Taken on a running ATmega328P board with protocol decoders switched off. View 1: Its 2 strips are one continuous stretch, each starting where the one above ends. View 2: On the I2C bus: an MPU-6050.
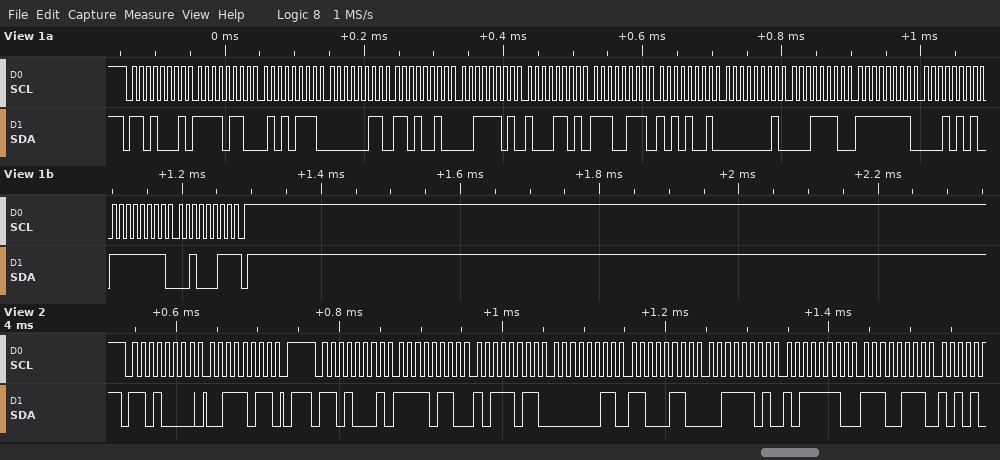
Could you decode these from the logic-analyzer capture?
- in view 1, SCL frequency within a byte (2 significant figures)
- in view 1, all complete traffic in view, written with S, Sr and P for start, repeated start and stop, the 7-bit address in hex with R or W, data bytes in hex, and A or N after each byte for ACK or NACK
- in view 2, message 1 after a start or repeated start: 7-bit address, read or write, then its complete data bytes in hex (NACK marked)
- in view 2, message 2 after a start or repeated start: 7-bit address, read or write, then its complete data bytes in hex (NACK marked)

100 kHz
S 68R A F6 A 57 A 03 A D2 A 3D A 8D A E7 A A9 A 01 A 1E A FF A 15 A FF A 23 N P
0x68 write: 3B
0x68 read: F6 BB 03 C6 3D BE E7
